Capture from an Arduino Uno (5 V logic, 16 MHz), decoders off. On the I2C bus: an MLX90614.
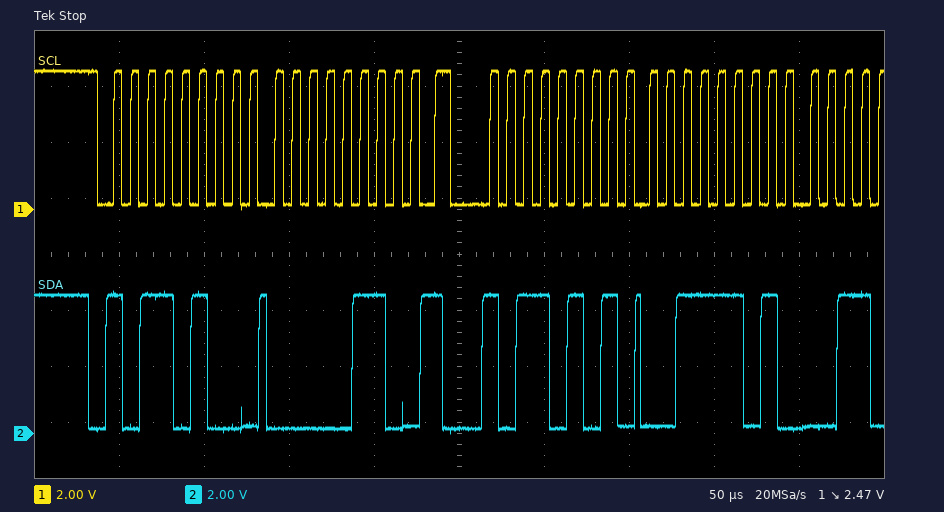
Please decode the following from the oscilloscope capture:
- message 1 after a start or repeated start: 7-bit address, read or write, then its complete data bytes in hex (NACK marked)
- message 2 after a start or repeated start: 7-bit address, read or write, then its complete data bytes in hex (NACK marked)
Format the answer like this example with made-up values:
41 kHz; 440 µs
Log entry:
0x5A write: 06; 0x5A read: 3D
